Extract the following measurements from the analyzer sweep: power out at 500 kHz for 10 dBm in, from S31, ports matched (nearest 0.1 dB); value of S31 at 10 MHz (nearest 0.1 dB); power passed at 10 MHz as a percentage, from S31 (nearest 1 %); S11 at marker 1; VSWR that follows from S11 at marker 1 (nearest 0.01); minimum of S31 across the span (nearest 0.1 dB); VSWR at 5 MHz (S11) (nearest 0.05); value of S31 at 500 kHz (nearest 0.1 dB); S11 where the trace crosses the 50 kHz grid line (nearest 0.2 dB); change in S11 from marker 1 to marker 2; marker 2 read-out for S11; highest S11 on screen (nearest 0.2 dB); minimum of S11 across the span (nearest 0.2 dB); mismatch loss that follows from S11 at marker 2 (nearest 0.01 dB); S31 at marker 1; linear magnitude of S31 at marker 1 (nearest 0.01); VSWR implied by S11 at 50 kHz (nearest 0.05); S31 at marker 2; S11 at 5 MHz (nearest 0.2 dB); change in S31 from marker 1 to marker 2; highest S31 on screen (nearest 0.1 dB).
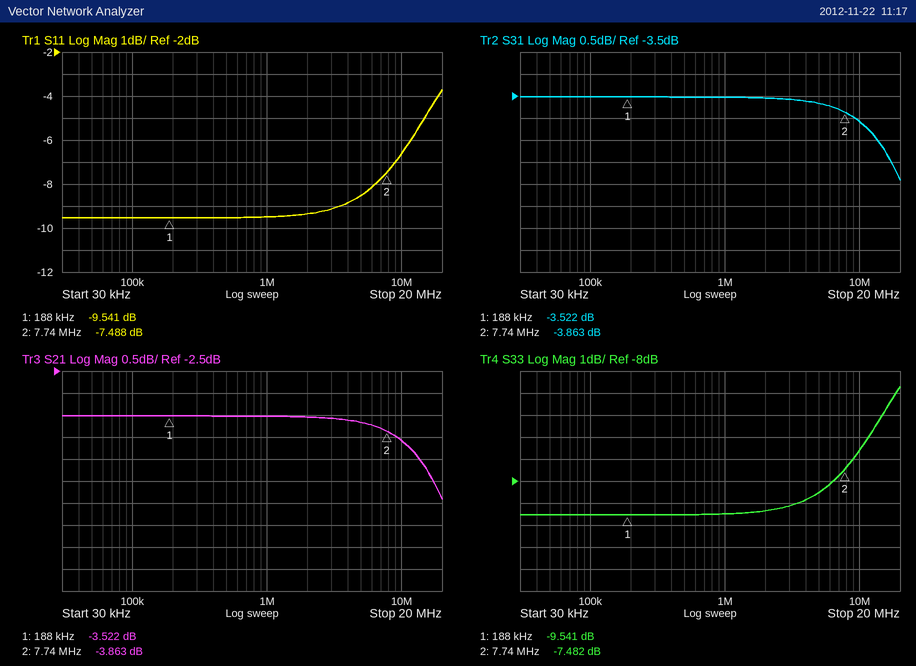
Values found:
6.5 dBm
-4.1 dB
39 %
-9.541 dB
2.00
-5.4 dB
2.20
-3.5 dB
-9.6 dB
2.053 dB
-7.488 dB
-3.8 dB
-9.6 dB
0.85 dB
-3.522 dB
0.67
2.00
-3.863 dB
-8.6 dB
-0.341 dB
-3.5 dB
